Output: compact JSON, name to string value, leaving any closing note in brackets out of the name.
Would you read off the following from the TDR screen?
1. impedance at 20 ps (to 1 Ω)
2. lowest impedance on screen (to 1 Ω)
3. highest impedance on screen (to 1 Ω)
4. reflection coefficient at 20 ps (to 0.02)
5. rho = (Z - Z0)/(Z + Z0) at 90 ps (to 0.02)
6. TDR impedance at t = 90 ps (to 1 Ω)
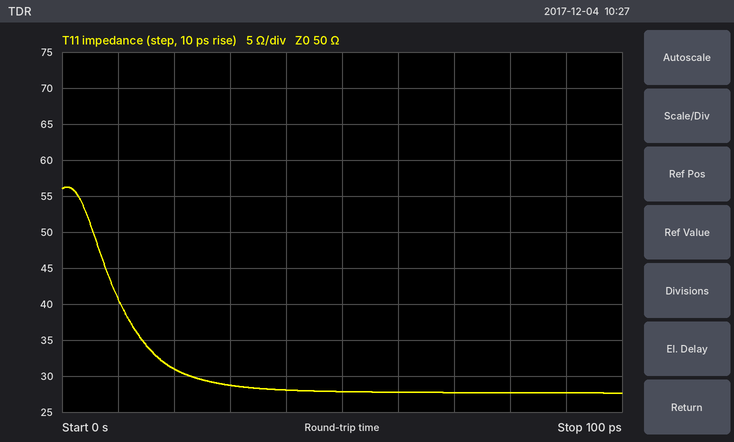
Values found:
{"impedance at 20 ps": "31 Ω", "lowest impedance on screen": "28 Ω", "highest impedance on screen": "56 Ω", "reflection coefficient at 20 ps": "-0.24", "rho = (Z - Z0)/(Z + Z0) at 90 ps": "-0.28", "TDR impedance at t = 90 ps": "28 Ω"}
